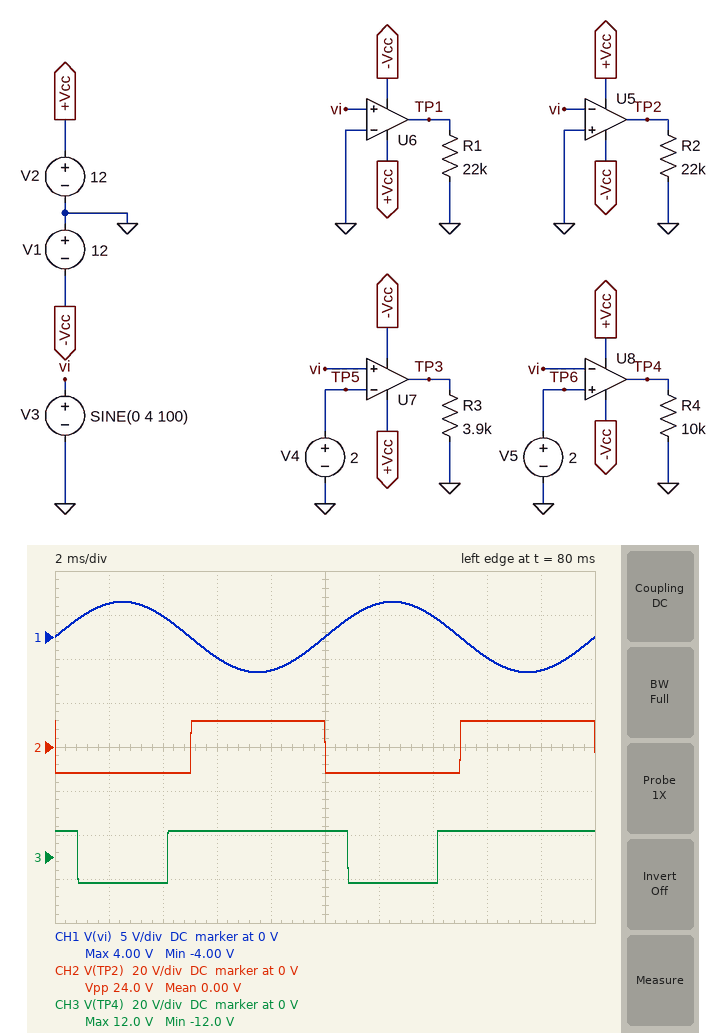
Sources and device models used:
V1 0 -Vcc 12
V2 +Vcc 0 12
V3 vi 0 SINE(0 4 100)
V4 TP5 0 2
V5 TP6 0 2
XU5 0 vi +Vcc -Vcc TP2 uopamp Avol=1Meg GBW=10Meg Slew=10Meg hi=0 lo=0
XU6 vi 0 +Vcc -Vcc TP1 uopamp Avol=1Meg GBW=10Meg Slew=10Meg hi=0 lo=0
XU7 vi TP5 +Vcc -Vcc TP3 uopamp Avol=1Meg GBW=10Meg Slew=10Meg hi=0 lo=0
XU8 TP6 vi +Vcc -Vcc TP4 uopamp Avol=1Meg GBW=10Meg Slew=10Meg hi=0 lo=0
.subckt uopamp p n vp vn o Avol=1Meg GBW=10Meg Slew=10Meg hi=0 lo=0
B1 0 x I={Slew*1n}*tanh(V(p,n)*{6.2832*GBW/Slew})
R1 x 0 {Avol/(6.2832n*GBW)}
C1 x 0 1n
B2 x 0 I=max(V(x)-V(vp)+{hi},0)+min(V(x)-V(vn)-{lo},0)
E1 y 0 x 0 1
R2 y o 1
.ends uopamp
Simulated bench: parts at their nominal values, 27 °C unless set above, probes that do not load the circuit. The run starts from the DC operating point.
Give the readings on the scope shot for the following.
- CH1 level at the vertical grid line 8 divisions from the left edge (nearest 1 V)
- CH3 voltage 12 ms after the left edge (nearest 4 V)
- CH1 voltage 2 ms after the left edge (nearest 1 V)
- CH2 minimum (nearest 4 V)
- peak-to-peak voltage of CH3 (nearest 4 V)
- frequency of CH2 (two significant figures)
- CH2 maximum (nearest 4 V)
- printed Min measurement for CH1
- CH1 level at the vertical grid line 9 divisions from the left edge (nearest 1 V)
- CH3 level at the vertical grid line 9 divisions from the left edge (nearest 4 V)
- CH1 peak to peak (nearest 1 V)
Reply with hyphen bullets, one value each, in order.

- -2 V
- -12 V
- 4 V
- -12 V
- 24 V
- 100 Hz
- 12 V
- -4.00 V
- -4 V
- 12 V
- 8 V
